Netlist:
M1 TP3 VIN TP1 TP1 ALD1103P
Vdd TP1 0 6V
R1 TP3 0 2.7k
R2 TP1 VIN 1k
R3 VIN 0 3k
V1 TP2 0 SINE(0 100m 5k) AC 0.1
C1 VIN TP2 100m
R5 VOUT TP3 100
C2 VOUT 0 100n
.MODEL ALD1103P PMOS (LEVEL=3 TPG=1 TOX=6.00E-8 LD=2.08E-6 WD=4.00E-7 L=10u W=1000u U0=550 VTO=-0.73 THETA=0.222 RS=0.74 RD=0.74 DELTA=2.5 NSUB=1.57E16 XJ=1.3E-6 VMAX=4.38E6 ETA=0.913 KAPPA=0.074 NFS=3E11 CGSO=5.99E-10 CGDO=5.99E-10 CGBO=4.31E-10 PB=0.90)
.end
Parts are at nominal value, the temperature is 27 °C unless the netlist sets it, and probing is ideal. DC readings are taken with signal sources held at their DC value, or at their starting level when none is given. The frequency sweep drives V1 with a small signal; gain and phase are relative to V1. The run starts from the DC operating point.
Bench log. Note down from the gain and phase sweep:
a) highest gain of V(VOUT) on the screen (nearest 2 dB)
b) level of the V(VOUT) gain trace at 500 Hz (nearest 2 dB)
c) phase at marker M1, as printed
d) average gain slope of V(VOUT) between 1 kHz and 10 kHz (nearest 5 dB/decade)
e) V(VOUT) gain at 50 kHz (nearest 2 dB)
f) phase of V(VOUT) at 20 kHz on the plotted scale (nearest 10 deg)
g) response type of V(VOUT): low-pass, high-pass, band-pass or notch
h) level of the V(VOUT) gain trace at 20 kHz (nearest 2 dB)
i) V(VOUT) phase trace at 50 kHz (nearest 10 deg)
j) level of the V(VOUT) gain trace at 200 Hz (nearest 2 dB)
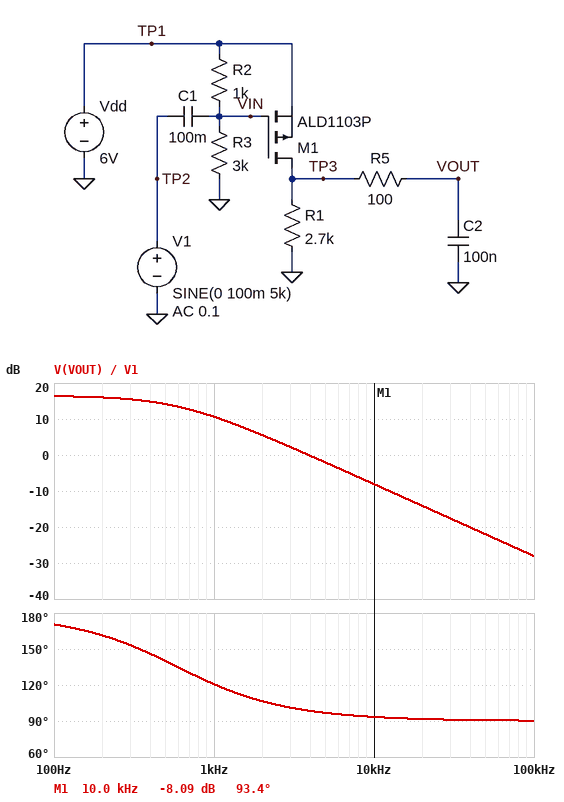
16 dB
14 dB
93.4 deg
-20 dB/decade
-22 dB
90 deg
low-pass
-14 dB
90 deg
16 dB
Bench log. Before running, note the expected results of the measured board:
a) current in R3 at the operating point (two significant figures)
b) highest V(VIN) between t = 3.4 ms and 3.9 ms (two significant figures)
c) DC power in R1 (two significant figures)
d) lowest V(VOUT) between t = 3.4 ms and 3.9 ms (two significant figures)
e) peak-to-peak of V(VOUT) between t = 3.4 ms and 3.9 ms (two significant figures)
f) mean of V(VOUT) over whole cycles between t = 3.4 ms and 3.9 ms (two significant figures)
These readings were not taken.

1.5 mA
4.6 V
3.7 mW
3.1 V
160 mV
3.2 V
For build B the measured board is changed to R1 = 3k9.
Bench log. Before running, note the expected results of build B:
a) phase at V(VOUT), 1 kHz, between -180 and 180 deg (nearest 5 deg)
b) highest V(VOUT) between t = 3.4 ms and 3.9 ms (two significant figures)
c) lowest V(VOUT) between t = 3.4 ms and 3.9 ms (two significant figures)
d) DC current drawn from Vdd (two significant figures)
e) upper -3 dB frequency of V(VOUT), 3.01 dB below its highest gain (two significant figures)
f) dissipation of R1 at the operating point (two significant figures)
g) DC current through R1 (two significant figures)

115 deg
4.6 V
4.4 V
2.6 mA
420 Hz
5.1 mW
1.1 mA
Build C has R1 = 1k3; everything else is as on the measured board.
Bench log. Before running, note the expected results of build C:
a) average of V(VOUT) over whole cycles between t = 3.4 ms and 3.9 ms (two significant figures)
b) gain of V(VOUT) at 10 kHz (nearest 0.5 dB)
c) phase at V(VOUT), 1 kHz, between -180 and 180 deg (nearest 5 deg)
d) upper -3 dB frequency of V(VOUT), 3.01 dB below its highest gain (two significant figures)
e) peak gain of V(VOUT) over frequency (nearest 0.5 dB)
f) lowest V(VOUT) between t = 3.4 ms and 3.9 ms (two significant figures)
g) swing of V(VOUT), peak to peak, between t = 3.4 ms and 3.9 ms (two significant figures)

1.6 V
-8.5 dB
140 deg
1.2 kHz
10.5 dB
1.5 V
150 mV
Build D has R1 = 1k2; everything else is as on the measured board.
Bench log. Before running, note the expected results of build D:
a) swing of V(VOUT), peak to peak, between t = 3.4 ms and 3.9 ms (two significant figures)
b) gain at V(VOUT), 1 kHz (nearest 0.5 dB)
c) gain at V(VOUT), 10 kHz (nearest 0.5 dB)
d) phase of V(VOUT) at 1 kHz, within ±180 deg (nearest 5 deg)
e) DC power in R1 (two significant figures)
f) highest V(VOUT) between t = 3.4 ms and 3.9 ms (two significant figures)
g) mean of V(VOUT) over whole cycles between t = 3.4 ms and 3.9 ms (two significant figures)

150 mV
7.5 dB
-8.5 dB
140 deg
1.7 mW
1.5 V
1.4 V
